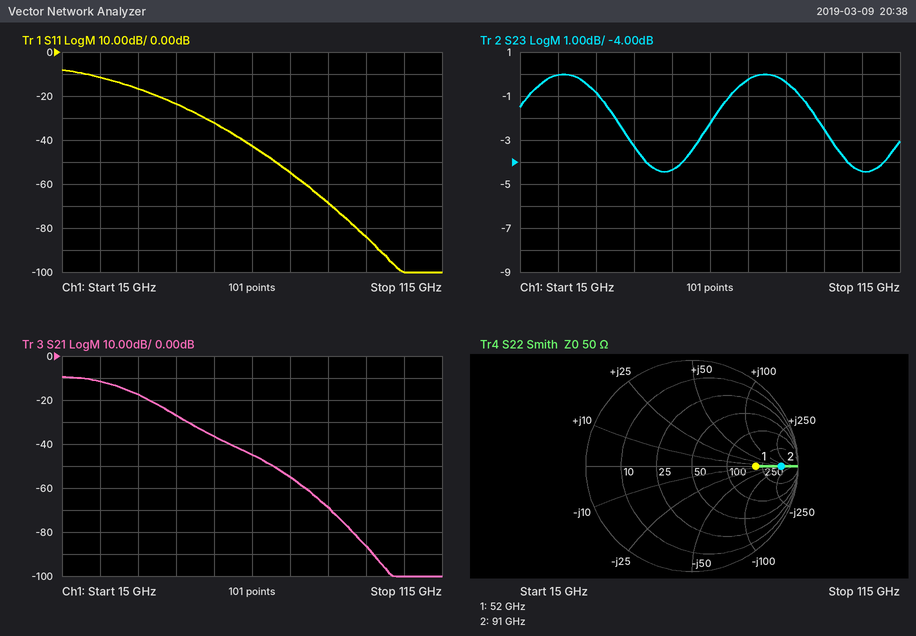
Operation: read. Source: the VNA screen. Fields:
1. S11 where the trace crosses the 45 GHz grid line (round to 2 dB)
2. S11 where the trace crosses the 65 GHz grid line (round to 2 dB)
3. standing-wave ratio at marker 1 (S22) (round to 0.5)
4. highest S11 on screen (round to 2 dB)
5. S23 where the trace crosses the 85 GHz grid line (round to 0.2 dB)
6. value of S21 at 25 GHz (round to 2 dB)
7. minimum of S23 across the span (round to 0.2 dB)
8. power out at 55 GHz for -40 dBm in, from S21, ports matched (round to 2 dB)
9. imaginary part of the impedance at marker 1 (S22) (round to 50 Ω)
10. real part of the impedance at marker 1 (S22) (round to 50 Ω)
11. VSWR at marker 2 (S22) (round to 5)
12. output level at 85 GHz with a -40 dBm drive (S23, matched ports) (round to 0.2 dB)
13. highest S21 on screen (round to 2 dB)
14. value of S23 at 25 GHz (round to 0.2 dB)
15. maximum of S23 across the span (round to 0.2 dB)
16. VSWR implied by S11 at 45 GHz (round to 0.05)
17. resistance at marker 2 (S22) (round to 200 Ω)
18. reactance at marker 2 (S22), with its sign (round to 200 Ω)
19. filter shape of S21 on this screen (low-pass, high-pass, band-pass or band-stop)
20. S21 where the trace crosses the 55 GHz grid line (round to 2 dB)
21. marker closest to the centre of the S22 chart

-24 dB
-42 dB
4.0
-8 dB
-0.4 dB
-12 dB
-4.4 dB
-76 dBm
0 Ω
200 Ω
10
-40.4 dBm
-10 dB
0.0 dB
0.0 dB
1.15
600 Ω
0 Ω
low-pass
-36 dB
marker 1
